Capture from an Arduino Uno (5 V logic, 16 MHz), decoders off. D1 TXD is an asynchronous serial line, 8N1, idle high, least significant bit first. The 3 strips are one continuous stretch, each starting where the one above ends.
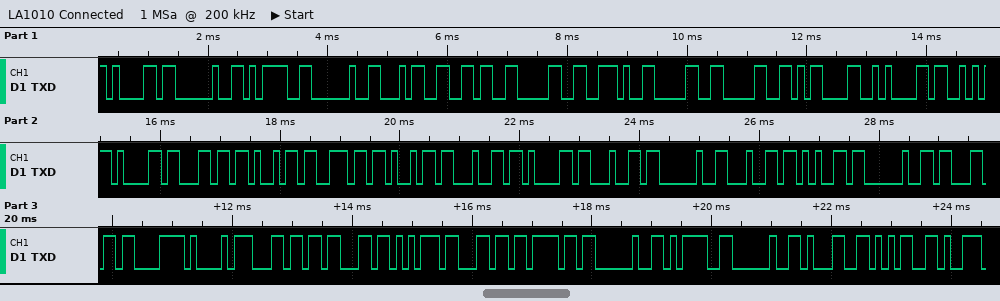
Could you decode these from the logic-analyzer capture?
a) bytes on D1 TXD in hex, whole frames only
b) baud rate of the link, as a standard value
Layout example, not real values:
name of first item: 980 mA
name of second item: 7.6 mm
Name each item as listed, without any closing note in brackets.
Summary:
bytes on D1 TXD in hex, whole frames only: 61 20 3D 20 34 36 30 2E 30 30 0D 0A 53 61 6C 69 6E 69 64 61 64 20 64 65 20 63 C3 A1 6C 63 75 6C 6F 20 3D 20 31 35
baud rate of the link, as a standard value: 9600 baud
